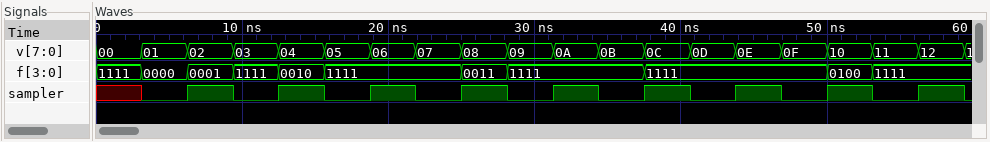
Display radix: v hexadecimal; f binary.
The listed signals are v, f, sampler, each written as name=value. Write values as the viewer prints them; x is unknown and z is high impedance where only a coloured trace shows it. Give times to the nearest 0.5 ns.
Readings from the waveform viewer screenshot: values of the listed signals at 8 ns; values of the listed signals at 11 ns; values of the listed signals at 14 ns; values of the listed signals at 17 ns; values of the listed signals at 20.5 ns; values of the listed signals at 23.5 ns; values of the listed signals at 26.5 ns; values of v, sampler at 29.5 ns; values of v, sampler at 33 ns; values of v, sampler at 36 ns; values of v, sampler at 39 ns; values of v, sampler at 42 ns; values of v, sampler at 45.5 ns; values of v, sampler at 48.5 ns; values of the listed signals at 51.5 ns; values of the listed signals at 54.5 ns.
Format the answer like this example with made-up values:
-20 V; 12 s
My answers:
v=02, f=0001, sampler=1; v=03, f=1111, sampler=0; v=04, f=0010, sampler=1; v=05, f=1111, sampler=0; v=06, f=1111, sampler=1; v=07, f=1111, sampler=0; v=08, f=0011, sampler=1; v=09, sampler=0; v=0A, sampler=1; v=0B, sampler=0; v=0C, sampler=1; v=0D, sampler=0; v=0E, sampler=1; v=0F, sampler=0; v=10, f=0100, sampler=1; v=11, f=1111, sampler=0
